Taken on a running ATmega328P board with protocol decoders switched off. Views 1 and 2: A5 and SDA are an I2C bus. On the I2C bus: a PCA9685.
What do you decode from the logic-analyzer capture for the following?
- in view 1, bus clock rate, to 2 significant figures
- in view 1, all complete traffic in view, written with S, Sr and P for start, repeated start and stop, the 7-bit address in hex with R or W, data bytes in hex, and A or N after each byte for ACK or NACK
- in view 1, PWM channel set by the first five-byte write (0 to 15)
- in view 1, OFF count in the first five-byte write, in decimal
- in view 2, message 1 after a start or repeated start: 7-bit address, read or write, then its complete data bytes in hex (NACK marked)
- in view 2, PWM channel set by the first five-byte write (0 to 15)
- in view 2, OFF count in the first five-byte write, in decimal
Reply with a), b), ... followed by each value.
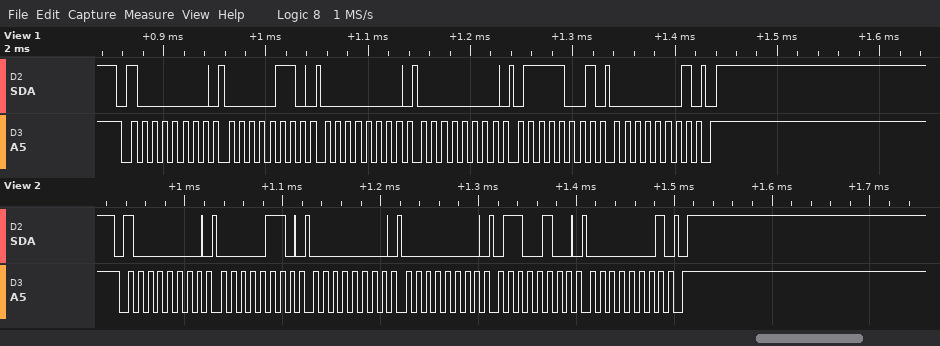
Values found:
a) 100 kHz
b) S 40W A 06 A 00 A 00 A 79 A 01 A P
c) 0
d) 377
e) 0x40 write: 06 00 00 64 01
f) 0
g) 356
